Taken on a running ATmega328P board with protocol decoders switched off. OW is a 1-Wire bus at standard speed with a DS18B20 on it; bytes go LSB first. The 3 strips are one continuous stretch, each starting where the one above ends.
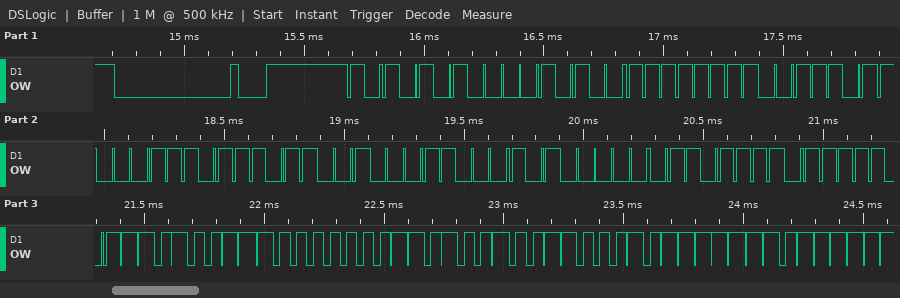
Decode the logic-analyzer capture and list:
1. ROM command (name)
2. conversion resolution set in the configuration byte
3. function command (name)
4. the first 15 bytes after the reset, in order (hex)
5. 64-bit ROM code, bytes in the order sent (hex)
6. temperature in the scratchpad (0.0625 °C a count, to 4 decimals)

Match ROM
12 bits
Read Scratchpad
55 28 FF DC B8 9B 18 05 F6 BE CB 01 4B 46 7F
28 FF DC B8 9B 18 05 F6
28.6875 °C
